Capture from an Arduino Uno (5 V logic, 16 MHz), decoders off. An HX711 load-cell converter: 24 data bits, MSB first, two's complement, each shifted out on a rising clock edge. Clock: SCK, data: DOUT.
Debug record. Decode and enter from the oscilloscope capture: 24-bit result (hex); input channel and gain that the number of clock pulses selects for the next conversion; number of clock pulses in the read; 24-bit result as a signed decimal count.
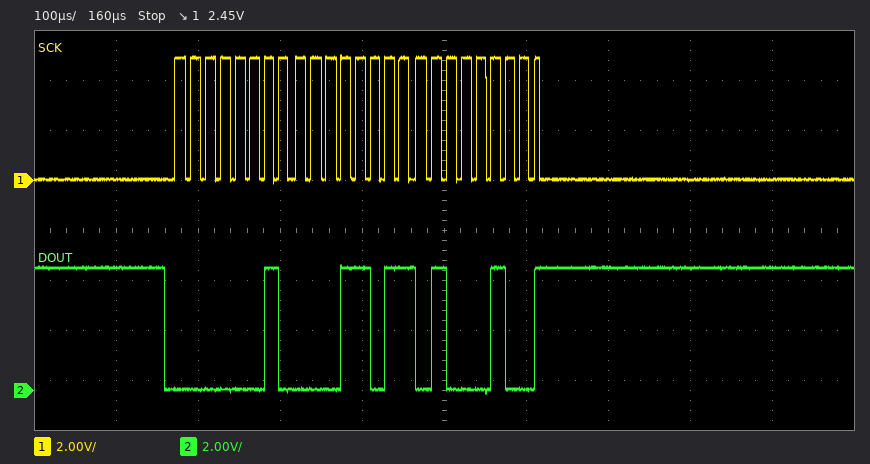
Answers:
0x021B44
channel A, gain 128
25
138052
